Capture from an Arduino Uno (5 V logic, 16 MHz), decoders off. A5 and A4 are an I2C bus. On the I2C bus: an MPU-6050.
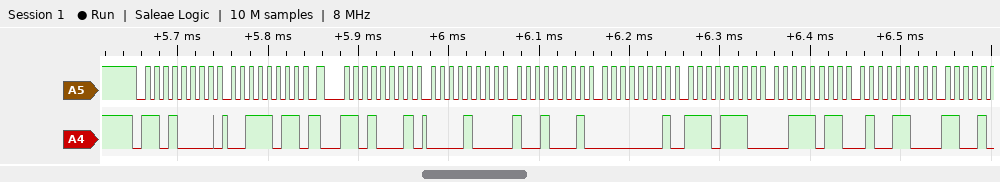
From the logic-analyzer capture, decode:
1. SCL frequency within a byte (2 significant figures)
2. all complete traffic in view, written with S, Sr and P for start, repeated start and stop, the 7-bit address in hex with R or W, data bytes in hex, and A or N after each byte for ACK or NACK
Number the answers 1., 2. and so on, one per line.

1. 100 kHz
2. S 68W A 3B A Sr 68R A 08 A 91 A 01 A EE A 3B A 4C A
